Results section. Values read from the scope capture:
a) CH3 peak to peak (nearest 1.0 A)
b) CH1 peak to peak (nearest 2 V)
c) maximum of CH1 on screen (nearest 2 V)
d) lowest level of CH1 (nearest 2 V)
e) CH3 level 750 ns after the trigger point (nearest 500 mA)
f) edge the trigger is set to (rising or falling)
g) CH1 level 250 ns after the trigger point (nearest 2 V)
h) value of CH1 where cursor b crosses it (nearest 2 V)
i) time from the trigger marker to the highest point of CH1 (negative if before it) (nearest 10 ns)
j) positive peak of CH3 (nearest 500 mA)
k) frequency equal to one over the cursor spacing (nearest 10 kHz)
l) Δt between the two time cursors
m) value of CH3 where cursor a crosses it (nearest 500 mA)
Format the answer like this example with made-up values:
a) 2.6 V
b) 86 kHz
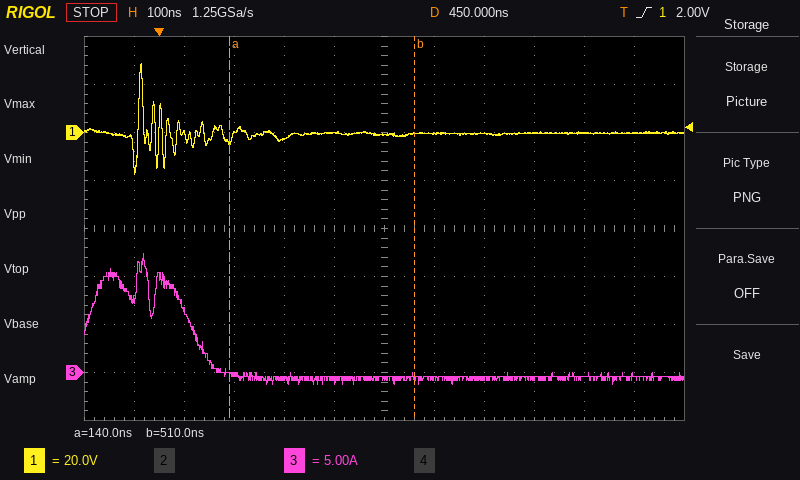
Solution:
a) 14.0 A
b) 46 V
c) 28 V
d) -18 V
e) -500 mA
f) rising
g) -2 V
h) 0 V
i) -40 ns
j) 12.5 A
k) 2.70 MHz
l) 370 ns
m) 0.0 A
